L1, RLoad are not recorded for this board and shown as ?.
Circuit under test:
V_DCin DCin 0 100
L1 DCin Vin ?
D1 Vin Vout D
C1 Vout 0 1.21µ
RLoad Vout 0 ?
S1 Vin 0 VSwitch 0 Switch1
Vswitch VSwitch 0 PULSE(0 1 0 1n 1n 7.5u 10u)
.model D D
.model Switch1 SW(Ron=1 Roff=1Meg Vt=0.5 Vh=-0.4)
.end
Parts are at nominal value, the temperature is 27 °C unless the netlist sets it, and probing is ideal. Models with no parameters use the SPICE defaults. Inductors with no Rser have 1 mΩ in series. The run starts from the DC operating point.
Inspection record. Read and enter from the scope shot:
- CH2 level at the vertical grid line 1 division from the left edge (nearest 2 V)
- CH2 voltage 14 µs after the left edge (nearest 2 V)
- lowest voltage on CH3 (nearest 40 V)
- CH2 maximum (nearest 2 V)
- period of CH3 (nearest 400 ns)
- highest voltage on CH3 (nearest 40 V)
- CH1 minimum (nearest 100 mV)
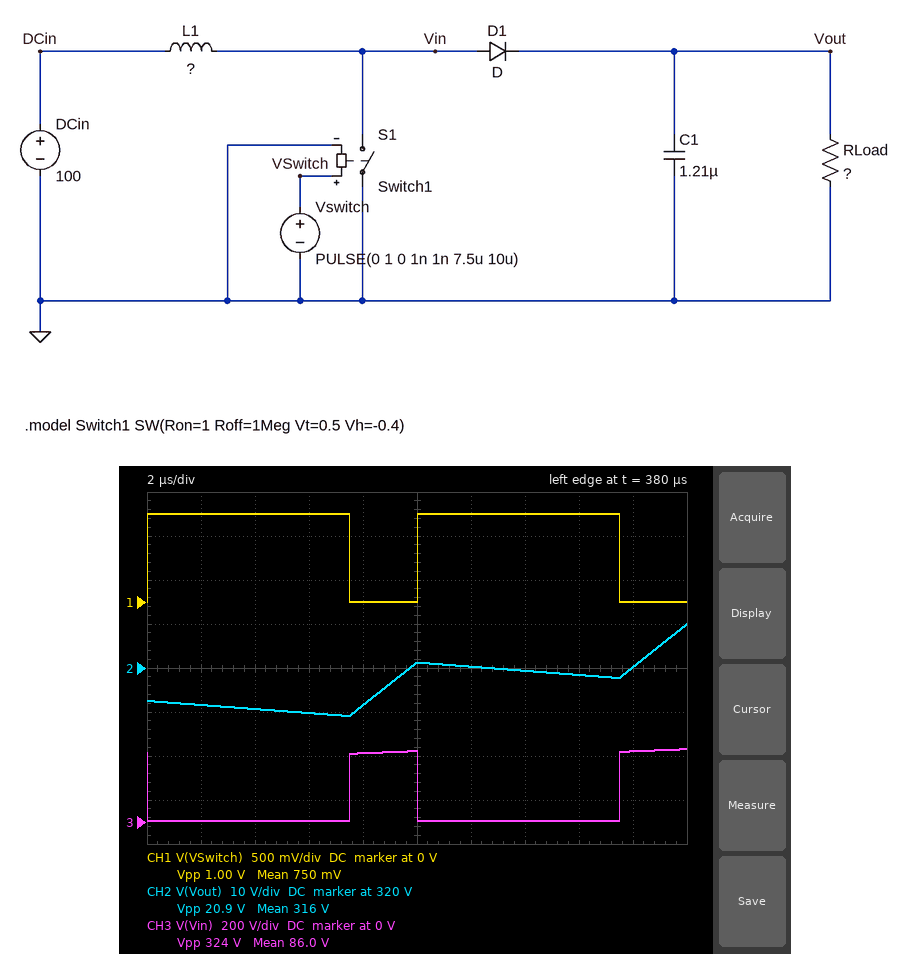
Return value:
312 V
320 V
0 V
330 V
10.0 µs
320 V
0 V
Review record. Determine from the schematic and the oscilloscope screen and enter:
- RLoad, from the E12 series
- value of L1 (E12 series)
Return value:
560 Ω
3.3 mH
